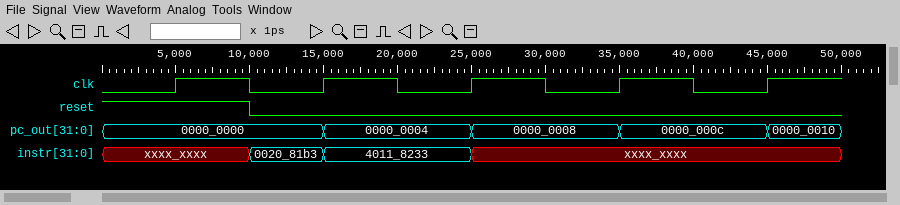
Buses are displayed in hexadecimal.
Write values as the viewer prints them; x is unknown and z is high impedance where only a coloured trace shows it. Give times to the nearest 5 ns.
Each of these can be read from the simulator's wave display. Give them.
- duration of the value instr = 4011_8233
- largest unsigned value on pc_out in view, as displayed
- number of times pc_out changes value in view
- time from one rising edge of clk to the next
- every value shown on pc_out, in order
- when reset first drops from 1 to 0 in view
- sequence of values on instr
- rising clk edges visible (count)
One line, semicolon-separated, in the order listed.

10 ns; 0000_0010; 4; 10 ns; 0000_0000, 0000_0004, 0000_0008, 0000_000c, 0000_0010; 10 ns; xxxx_xxxx, 0020_81b3, 4011_8233, xxxx_xxxx; 5
